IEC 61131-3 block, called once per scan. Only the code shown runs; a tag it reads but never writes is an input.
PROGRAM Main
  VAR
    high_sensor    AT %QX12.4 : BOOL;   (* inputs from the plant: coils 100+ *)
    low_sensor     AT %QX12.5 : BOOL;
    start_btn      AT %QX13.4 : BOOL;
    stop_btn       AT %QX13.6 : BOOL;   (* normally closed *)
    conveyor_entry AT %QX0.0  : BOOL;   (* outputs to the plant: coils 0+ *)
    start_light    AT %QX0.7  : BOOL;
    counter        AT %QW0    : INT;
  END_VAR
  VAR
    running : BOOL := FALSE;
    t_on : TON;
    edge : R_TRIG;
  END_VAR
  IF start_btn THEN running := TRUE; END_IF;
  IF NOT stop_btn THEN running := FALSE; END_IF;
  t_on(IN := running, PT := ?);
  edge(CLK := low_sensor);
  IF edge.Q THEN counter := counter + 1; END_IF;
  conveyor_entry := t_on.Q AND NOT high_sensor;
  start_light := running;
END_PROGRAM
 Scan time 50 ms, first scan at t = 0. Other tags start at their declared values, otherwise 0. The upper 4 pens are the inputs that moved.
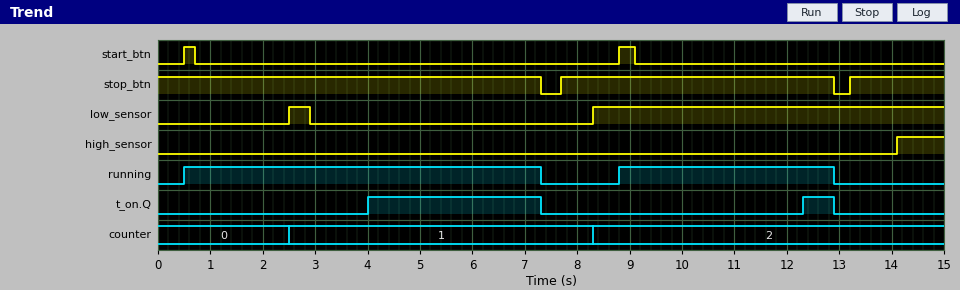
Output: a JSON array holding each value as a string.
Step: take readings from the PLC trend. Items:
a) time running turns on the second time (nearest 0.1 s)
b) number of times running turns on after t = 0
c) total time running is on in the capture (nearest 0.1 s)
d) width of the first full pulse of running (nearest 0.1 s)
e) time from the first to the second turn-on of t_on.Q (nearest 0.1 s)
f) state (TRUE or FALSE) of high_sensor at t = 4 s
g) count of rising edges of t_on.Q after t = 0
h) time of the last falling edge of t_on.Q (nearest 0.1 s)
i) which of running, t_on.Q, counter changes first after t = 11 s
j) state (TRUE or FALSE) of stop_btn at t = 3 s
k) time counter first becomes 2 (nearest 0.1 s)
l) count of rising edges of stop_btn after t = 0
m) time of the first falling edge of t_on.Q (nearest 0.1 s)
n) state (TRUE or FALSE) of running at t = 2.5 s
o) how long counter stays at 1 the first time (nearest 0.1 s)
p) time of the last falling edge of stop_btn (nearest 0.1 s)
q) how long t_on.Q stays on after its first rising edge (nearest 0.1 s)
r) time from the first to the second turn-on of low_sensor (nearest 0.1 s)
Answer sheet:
["8.8 s", "2", "10.9 s", "6.8 s", "8.3 s", "FALSE", "2", "12.9 s", "t_on.Q", "TRUE", "8.3 s", "2", "7.3 s", "TRUE", "5.8 s", "12.9 s", "3.3 s", "5.8 s"]
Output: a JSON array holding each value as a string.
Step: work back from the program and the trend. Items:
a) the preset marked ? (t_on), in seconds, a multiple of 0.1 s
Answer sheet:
["3.5 s"]
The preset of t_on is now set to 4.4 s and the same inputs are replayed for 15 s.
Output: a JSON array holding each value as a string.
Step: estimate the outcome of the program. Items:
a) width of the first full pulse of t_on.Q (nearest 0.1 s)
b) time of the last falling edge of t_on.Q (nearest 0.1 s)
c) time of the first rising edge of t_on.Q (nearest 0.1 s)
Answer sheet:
["2.4 s", "7.3 s", "4.9 s"]
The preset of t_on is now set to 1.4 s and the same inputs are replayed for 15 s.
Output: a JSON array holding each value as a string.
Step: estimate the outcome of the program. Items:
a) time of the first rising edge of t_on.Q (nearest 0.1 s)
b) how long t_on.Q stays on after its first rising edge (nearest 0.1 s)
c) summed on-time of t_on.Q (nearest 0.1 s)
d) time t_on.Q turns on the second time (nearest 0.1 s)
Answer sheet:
["1.9 s", "5.4 s", "8.1 s", "10.2 s"]
